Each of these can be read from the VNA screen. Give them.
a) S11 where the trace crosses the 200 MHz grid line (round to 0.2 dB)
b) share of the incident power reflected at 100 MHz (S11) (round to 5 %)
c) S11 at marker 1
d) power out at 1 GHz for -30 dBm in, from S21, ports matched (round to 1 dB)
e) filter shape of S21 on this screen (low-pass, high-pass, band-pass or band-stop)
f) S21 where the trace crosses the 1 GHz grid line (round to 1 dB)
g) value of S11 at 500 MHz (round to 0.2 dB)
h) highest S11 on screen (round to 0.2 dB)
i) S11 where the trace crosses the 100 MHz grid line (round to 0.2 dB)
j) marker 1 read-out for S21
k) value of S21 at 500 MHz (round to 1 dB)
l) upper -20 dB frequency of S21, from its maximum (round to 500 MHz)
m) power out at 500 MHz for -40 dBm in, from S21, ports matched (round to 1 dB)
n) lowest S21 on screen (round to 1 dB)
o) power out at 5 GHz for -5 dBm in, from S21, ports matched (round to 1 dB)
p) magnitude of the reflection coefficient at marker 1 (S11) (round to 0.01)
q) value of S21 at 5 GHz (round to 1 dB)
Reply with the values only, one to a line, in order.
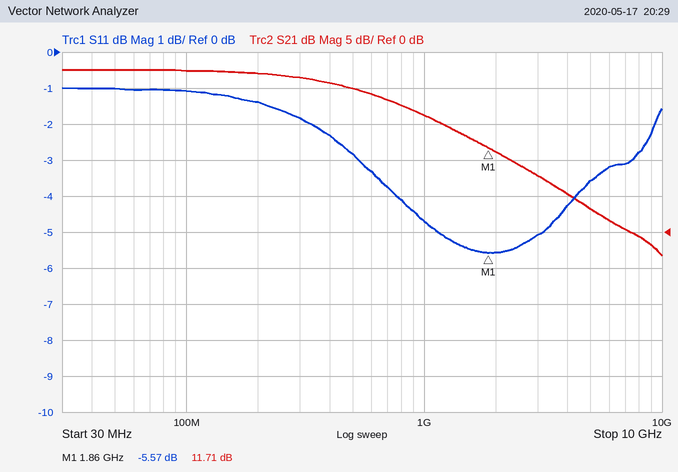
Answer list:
-1.4 dB
80 %
-5.57 dB
-14 dBm
low-pass
16 dB
-2.8 dB
-1.0 dB
-1.0 dB
11.71 dB
20 dB
5.5 GHz
-20 dBm
-3 dB
-2 dBm
0.53
3 dB
